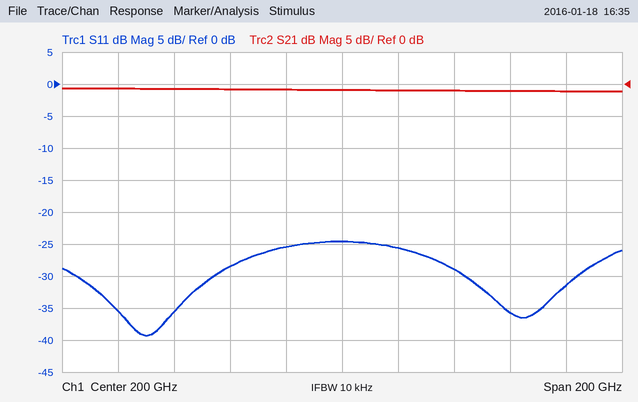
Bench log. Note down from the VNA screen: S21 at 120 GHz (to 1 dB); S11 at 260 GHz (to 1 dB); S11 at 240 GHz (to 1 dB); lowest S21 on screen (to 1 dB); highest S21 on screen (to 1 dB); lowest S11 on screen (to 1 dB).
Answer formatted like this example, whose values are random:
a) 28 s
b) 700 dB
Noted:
a) -1 dB
b) -36 dB
c) -29 dB
d) -1 dB
e) -1 dB
f) -39 dB
